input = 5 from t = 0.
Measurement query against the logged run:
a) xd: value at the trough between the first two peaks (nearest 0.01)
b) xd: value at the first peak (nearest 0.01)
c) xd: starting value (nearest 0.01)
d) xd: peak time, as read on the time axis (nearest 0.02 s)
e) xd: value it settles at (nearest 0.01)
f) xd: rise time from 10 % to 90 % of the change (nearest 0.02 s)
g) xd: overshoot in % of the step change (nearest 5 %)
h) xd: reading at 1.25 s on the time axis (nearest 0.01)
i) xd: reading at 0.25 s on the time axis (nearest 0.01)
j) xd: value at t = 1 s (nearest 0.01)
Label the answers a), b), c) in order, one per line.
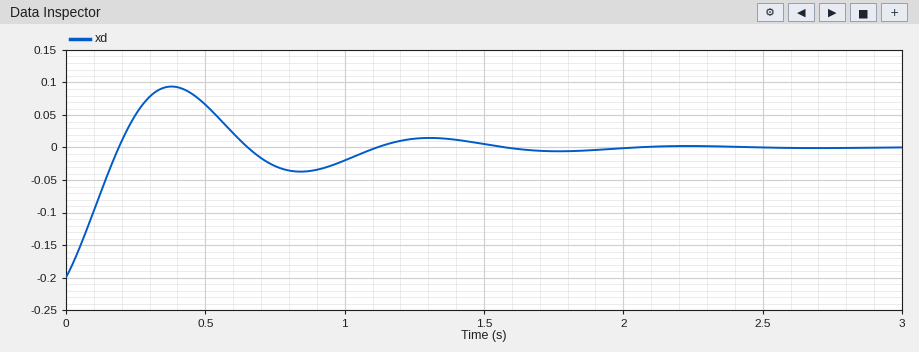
a) -0.04
b) 0.09
c) -0.20
d) 0.38 s
e) 0.00
f) 0.14 s
g) 45 %
h) 0.01
i) 0.05
j) -0.02
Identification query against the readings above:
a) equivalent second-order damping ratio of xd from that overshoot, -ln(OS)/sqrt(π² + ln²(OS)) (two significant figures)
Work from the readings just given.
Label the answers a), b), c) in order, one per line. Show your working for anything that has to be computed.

a) ln(0.45) = -0.799; 0.799 / sqrt(9.870 + 0.638) = 0.25
